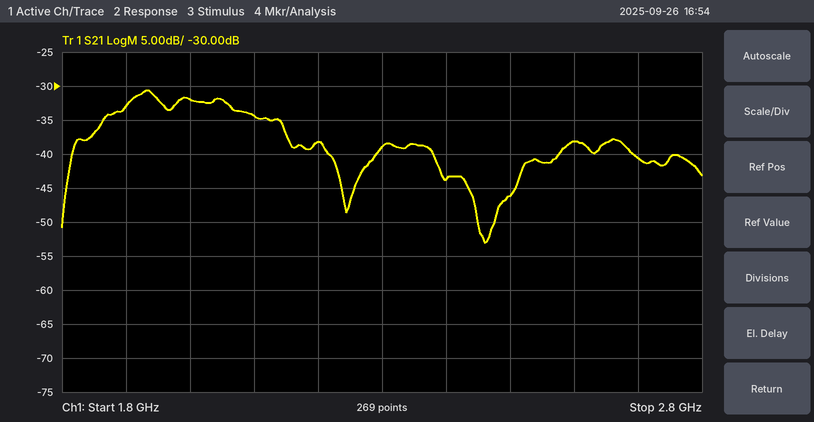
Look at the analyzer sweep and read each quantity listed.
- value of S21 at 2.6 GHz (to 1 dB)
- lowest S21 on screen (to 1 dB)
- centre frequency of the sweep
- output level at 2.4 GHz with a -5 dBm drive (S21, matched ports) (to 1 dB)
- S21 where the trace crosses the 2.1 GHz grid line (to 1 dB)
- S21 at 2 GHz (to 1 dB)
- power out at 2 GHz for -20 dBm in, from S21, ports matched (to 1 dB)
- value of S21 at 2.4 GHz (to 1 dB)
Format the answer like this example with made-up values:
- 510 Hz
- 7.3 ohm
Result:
- -38 dB
- -53 dB
- 2.3 GHz
- -49 dBm
- -34 dB
- -32 dB
- -52 dBm
- -44 dB
